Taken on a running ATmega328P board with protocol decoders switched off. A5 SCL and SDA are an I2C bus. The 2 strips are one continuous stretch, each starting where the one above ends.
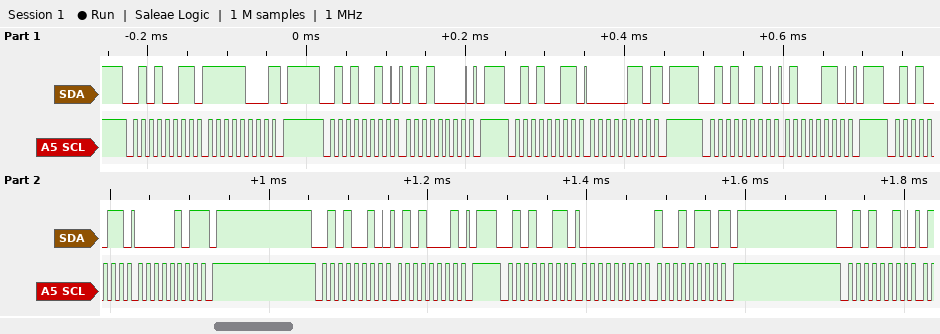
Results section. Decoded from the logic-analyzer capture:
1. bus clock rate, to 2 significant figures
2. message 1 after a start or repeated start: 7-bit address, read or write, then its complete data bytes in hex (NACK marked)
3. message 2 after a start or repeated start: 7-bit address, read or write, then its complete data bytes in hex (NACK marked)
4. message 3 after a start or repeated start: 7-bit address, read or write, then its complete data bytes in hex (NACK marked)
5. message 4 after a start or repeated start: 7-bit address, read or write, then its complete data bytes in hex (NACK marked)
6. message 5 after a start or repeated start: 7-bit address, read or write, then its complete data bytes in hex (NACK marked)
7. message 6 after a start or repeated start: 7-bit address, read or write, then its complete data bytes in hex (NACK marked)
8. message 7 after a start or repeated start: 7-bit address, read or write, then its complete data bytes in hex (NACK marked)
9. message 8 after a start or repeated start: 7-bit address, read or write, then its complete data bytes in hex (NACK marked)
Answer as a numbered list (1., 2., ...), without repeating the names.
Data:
1. 100 kHz
2. 0x29 read: F8 NACK
3. 0x29 write: 50
4. 0x29 read: 06 NACK
5. 0x29 write: 46
6. 0x29 read: 05 NACK
7. 0x29 write: 51
8. 0x29 read: 00 96 NACK
9. 0x29 write
